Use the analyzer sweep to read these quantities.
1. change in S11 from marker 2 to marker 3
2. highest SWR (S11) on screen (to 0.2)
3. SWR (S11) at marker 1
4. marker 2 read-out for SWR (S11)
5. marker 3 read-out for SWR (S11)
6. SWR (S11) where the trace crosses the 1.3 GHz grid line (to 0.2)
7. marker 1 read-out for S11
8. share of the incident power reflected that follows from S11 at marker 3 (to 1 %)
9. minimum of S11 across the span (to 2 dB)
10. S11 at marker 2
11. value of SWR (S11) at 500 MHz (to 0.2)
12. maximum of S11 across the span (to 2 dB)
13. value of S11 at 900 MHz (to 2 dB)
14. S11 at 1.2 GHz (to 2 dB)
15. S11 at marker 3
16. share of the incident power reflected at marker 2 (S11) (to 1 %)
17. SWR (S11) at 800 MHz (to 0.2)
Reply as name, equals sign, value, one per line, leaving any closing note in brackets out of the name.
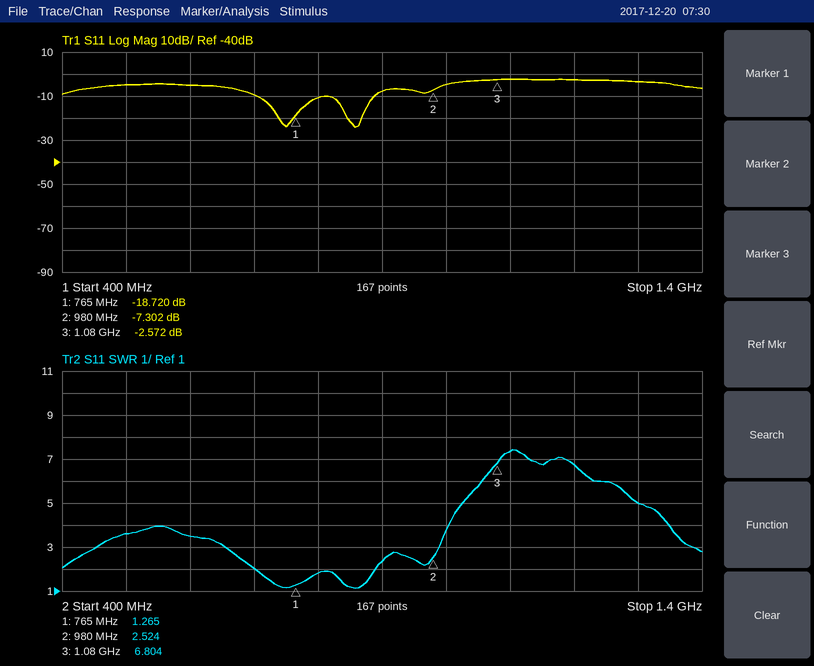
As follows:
change in S11 from marker 2 to marker 3 = 4.730 dB
highest SWR (S11) on screen = 7.4
SWR (S11) at marker 1 = 1.265
marker 2 read-out for SWR = 2.524
marker 3 read-out for SWR = 6.804
SWR (S11) where the trace crosses the 1.3 GHz grid line = 5.0
marker 1 read-out for S11 = -18.720 dB
share of the incident power reflected that follows from S11 at marker 3 = 55 %
minimum of S11 across the span = -24 dB
S11 at marker 2 = -7.302 dB
value of SWR (S11) at 500 MHz = 3.6
maximum of S11 across the span = -2 dB
value of S11 at 900 MHz = -8 dB
S11 at 1.2 GHz = -2 dB
S11 at marker 3 = -2.572 dB
share of the incident power reflected at marker 2 (S11) = 19 %
SWR (S11) at 800 MHz = 1.8
